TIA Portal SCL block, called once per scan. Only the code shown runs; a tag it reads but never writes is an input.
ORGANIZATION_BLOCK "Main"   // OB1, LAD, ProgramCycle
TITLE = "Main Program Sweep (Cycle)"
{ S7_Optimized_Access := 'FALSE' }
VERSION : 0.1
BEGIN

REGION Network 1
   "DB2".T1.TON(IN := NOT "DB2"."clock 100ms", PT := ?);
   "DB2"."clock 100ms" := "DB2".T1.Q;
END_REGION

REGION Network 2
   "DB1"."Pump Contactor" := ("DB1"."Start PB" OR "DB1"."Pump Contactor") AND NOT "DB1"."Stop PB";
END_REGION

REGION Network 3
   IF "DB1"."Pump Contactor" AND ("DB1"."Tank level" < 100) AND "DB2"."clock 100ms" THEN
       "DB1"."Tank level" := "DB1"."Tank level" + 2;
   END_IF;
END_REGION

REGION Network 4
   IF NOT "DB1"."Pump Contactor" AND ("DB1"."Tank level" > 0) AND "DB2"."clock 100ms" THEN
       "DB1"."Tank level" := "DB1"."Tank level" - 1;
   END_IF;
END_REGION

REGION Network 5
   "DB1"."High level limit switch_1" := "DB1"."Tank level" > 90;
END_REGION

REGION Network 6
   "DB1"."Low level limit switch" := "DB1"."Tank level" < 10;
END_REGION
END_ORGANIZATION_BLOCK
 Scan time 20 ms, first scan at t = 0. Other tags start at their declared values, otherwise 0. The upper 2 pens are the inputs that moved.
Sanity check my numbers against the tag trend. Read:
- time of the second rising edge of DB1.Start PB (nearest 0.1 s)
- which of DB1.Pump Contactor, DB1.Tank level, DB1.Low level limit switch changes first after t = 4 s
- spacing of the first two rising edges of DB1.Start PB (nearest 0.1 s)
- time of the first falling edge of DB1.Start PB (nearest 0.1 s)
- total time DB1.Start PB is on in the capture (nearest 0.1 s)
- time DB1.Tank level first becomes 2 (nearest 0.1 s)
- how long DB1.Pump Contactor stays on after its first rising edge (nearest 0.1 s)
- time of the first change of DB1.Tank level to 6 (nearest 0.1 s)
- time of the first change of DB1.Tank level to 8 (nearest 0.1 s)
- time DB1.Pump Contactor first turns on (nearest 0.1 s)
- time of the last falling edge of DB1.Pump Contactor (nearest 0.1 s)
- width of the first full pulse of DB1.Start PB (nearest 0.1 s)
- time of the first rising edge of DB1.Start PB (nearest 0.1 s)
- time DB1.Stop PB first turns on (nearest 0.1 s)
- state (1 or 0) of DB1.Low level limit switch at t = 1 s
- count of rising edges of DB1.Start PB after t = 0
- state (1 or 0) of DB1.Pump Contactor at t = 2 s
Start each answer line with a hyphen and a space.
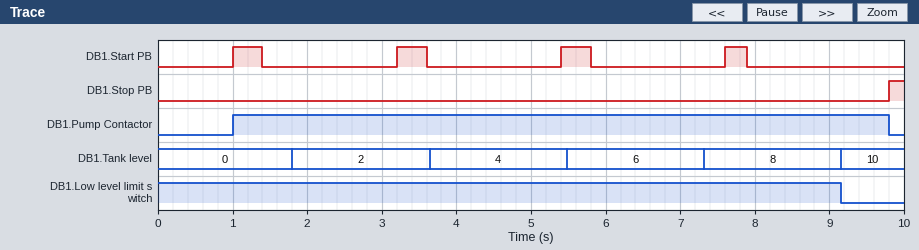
- 3.2 s
- DB1.Tank level
- 2.2 s
- 1.4 s
- 1.5 s
- 1.8 s
- 8.8 s
- 5.5 s
- 7.3 s
- 1.0 s
- 9.8 s
- 0.4 s
- 1.0 s
- 9.8 s
- 1
- 4
- 1
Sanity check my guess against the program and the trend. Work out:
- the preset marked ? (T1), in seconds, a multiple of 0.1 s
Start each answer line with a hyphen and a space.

- 1.8 s
